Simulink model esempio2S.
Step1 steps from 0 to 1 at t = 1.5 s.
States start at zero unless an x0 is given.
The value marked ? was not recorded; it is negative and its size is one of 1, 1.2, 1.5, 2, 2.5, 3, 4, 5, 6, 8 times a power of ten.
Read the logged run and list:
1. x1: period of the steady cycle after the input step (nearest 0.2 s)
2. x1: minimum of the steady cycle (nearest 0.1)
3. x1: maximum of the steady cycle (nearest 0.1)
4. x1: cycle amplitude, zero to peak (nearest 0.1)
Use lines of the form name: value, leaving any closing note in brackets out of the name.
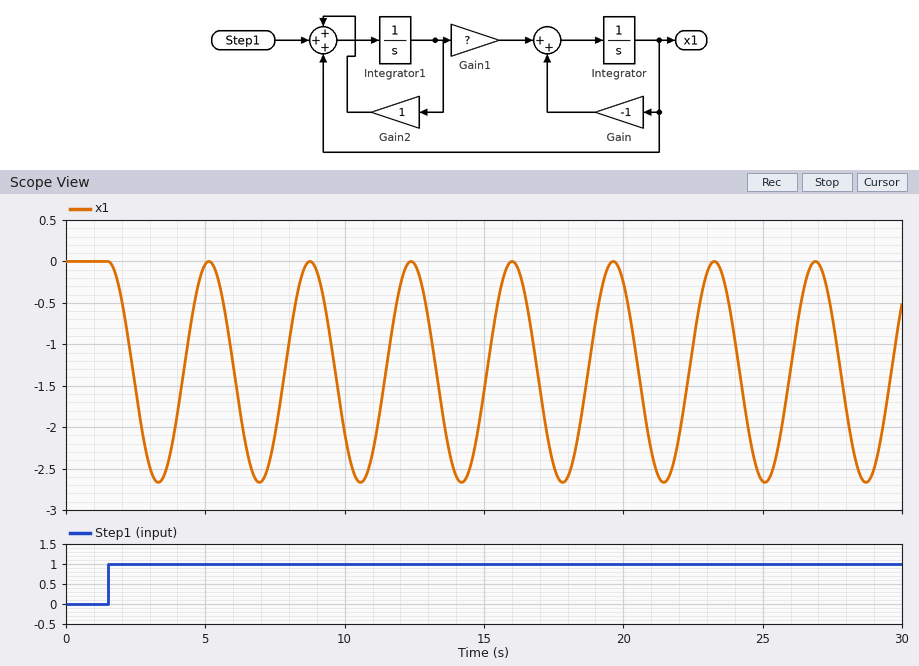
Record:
x1: period of the steady cycle after the input step: 3.6 s
x1: minimum of the steady cycle: -2.7
x1: maximum of the steady cycle: 0.0
x1: cycle amplitude, zero to peak: 1.3
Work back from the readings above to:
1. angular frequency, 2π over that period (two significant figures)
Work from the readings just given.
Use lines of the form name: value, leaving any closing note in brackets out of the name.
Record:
angular frequency, 2π over that period: 1.7 rad/s
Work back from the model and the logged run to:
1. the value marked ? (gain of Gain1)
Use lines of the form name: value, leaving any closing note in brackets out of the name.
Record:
the value marked ?: -4
